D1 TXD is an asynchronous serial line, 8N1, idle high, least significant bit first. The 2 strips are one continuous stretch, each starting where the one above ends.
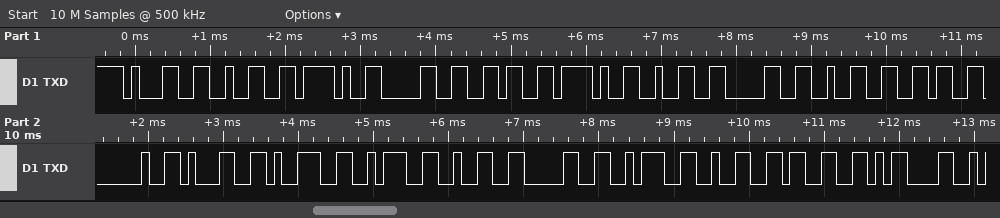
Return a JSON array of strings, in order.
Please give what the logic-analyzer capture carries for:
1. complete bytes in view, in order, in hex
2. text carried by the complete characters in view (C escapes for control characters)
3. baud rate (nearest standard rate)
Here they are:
["31 32 2F 30 36 2F 32 30 32 36 20 31 39 3A 32 30 3A 32 33 0D", "\"12/06/2026 19:20:23\\r\"", "9600 baud"]
